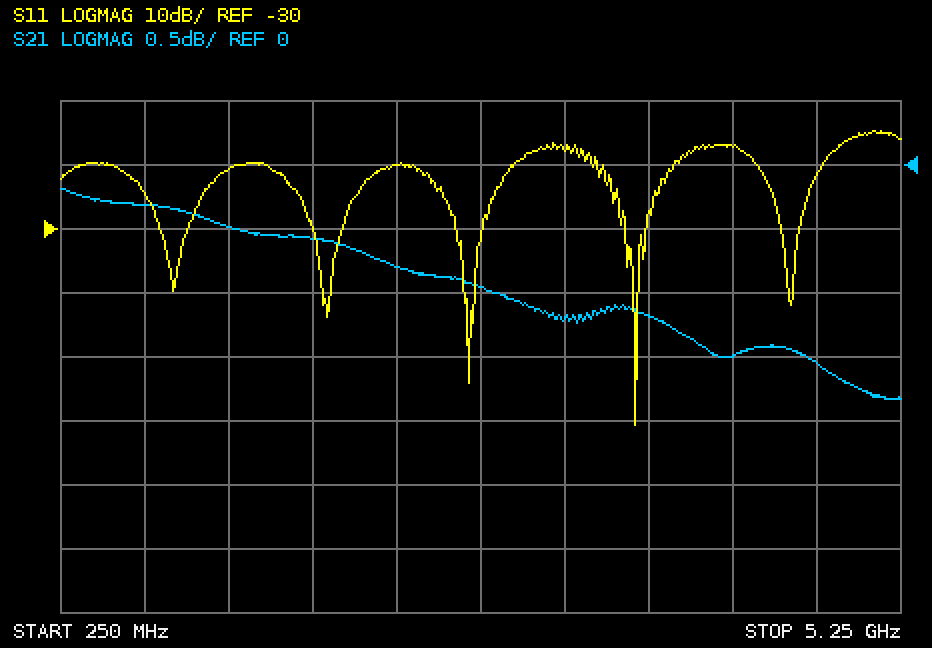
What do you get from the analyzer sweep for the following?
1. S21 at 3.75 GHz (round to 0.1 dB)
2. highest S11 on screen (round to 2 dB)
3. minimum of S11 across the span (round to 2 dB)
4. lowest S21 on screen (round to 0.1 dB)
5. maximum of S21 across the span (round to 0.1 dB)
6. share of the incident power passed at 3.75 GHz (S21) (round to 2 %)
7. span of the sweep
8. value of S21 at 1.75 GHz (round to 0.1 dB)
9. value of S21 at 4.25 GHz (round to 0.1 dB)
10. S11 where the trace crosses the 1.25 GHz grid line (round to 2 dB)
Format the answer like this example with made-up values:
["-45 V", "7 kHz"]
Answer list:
["-1.2 dB", "-14 dB", "-60 dB", "-1.8 dB", "-0.2 dB", "76 %", "5 GHz", "-0.6 dB", "-1.5 dB", "-20 dB"]
